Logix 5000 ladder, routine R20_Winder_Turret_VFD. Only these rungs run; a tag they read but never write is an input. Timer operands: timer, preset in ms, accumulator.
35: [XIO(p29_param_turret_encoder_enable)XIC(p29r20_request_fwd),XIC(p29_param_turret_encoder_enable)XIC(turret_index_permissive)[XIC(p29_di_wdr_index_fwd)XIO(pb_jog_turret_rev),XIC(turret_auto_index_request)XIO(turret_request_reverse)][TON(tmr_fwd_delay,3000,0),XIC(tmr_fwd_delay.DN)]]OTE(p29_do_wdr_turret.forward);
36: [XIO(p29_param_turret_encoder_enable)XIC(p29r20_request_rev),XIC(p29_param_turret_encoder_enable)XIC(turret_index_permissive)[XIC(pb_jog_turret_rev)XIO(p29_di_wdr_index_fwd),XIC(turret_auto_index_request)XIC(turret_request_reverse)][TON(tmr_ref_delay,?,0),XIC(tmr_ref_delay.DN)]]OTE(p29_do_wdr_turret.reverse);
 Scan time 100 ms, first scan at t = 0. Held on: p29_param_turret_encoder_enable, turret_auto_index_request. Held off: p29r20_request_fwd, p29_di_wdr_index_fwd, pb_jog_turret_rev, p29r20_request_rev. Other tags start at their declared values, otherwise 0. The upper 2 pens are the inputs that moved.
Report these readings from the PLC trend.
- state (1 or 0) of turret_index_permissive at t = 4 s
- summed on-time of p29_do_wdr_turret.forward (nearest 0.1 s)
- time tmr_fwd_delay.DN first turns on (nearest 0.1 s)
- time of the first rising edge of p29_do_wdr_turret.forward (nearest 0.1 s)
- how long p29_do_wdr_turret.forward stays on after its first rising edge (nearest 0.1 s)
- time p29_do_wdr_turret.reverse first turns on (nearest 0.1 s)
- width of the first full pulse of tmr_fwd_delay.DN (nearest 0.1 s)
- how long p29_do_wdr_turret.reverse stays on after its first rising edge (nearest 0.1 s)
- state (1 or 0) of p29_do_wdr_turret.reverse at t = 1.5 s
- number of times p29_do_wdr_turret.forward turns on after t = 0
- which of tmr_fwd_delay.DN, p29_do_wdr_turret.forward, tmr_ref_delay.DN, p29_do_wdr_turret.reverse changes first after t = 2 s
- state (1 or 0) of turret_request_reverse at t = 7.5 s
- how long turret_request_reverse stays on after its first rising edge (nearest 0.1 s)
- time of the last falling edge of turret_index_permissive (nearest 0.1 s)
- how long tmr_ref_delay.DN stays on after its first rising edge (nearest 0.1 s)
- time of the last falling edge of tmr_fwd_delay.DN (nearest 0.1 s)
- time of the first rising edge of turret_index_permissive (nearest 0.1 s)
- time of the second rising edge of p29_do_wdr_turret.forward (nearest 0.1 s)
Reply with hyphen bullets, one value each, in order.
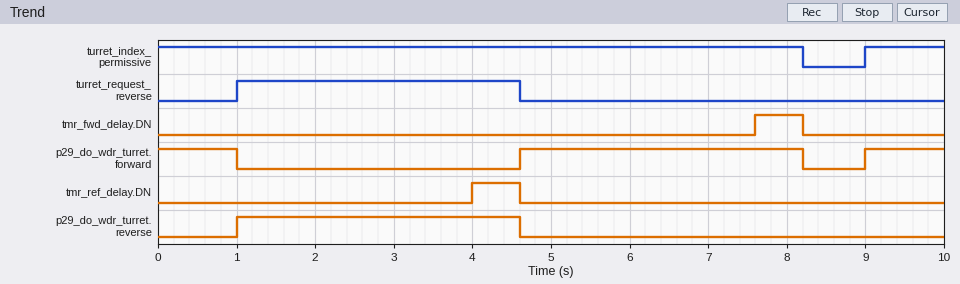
- 1
- 5.6 s
- 7.6 s
- 4.6 s
- 3.6 s
- 1.0 s
- 0.6 s
- 3.6 s
- 1
- 2
- tmr_ref_delay.DN
- 0
- 3.6 s
- 8.2 s
- 0.6 s
- 8.2 s
- 9.0 s
- 9.0 s
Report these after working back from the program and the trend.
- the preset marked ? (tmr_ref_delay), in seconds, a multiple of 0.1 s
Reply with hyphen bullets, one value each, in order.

- 3.0 s
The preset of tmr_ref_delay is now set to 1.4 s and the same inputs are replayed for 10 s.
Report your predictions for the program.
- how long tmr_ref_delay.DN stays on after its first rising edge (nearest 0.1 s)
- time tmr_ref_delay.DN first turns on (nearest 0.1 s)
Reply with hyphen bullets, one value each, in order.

- 2.2 s
- 2.4 s
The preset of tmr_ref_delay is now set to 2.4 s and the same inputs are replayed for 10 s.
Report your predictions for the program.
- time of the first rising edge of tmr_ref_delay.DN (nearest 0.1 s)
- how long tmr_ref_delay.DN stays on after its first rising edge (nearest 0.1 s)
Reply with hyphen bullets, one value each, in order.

- 3.4 s
- 1.2 s
